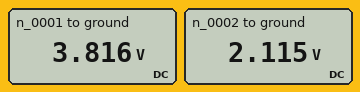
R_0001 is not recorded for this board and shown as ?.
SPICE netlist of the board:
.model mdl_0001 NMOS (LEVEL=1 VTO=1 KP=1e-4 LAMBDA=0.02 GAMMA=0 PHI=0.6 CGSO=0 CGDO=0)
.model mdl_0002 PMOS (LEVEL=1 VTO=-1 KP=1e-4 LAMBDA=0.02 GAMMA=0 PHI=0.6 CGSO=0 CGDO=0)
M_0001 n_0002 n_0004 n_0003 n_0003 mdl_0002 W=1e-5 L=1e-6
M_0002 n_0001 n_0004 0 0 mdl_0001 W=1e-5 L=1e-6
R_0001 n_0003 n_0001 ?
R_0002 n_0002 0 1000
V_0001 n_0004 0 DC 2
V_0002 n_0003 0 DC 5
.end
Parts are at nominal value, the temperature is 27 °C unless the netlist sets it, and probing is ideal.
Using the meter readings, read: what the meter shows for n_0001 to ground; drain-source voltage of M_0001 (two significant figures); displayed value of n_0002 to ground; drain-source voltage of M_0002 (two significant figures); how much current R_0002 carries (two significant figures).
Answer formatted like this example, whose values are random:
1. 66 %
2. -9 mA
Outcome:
1. 3.816 V
2. -2.9 V
3. 2.115 V
4. 3.8 V
5. 2.1 mA
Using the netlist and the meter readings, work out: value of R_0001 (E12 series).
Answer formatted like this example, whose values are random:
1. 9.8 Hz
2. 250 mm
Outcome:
1. 2.2 kΩ
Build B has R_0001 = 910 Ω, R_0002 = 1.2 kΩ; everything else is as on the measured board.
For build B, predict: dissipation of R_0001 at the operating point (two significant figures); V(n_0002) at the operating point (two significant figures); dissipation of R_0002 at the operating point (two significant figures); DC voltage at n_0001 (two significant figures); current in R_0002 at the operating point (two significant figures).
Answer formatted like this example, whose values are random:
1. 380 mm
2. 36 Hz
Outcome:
1. 270 µW
2. 2.5 V
3. 5.3 mW
4. 4.5 V
5. 2.1 mA
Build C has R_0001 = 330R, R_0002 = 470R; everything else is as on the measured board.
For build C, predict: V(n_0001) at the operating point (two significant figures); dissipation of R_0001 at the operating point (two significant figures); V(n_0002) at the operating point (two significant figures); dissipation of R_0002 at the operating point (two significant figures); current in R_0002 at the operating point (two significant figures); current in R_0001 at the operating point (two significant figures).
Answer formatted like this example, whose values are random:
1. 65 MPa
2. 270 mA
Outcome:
1. 4.8 V
2. 99 µW
3. 1.0 V
4. 2.2 mW
5. 2.2 mA
6. 550 µA
